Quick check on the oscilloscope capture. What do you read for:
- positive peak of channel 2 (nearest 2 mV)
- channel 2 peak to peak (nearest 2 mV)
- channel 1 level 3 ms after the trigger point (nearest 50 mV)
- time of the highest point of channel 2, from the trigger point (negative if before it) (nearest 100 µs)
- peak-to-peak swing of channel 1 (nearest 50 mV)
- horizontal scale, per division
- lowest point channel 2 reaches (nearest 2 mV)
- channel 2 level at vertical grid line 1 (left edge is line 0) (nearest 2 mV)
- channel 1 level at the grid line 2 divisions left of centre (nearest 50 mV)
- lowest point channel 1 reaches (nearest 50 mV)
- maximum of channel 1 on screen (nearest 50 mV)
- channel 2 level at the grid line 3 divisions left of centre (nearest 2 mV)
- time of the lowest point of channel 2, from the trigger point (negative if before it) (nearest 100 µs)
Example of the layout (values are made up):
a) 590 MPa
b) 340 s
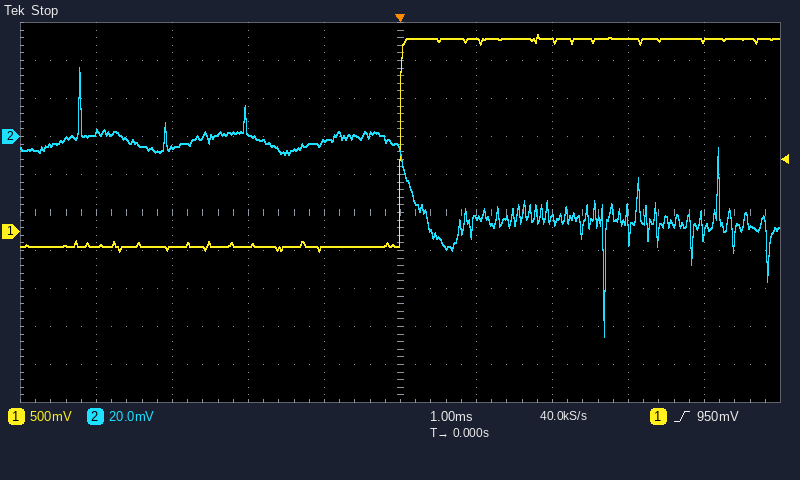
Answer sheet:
a) 36 mV
b) 142 mV
c) 2.55 V
d) -4.2 ms
e) 2.85 V
f) 1 ms
g) -106 mV
h) 2 mV
i) -200 mV
j) -250 mV
k) 2.60 V
l) -6 mV
m) +2.7 ms
